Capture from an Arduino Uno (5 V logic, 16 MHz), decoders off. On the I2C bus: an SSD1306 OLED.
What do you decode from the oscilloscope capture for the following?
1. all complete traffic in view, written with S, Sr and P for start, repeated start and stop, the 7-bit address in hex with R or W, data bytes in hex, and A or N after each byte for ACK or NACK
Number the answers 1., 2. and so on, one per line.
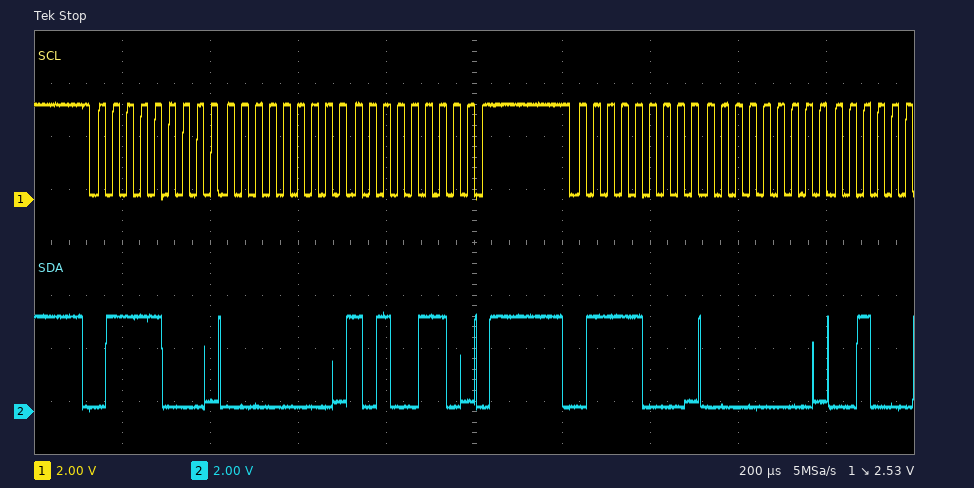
1. S 3CW A 00 A A6 A P S 3CW A 00 A
